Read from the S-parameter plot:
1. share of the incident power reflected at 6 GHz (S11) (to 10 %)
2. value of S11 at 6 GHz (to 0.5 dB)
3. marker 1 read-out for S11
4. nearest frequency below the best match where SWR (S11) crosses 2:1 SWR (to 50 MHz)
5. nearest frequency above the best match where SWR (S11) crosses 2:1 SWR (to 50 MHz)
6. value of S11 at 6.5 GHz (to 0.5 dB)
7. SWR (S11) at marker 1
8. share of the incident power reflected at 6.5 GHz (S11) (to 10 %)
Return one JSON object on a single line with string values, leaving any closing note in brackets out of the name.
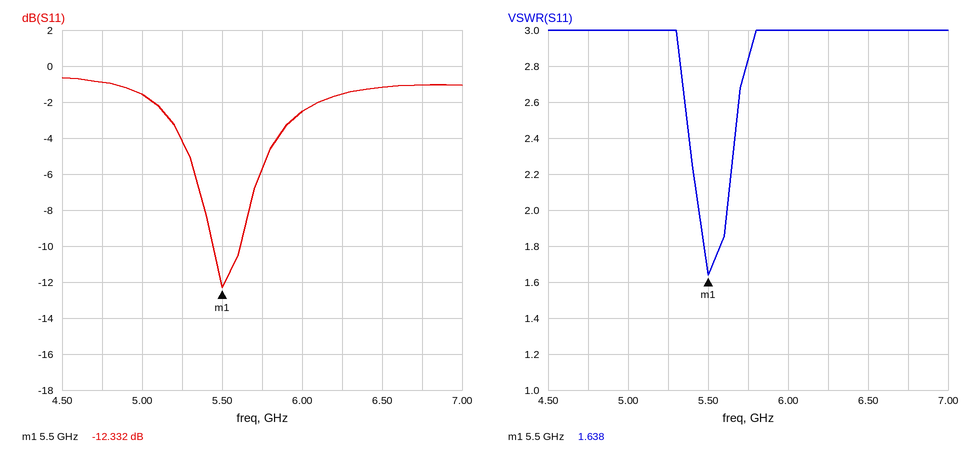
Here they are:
{"share of the incident power reflected at 6 GHz (S11)": "60 %", "value of S11 at 6 GHz": "-2.5 dB", "marker 1 read-out for S11": "-12.332 dB", "nearest frequency below the best match where SWR (S11) crosses 2:1 SWR": "5.45 GHz", "nearest frequency above the best match where SWR (S11) crosses 2:1 SWR": "5.60 GHz", "value of S11 at 6.5 GHz": "-1.0 dB", "SWR (S11) at marker 1": "1.638", "share of the incident power reflected at 6.5 GHz (S11)": "80 %"}
